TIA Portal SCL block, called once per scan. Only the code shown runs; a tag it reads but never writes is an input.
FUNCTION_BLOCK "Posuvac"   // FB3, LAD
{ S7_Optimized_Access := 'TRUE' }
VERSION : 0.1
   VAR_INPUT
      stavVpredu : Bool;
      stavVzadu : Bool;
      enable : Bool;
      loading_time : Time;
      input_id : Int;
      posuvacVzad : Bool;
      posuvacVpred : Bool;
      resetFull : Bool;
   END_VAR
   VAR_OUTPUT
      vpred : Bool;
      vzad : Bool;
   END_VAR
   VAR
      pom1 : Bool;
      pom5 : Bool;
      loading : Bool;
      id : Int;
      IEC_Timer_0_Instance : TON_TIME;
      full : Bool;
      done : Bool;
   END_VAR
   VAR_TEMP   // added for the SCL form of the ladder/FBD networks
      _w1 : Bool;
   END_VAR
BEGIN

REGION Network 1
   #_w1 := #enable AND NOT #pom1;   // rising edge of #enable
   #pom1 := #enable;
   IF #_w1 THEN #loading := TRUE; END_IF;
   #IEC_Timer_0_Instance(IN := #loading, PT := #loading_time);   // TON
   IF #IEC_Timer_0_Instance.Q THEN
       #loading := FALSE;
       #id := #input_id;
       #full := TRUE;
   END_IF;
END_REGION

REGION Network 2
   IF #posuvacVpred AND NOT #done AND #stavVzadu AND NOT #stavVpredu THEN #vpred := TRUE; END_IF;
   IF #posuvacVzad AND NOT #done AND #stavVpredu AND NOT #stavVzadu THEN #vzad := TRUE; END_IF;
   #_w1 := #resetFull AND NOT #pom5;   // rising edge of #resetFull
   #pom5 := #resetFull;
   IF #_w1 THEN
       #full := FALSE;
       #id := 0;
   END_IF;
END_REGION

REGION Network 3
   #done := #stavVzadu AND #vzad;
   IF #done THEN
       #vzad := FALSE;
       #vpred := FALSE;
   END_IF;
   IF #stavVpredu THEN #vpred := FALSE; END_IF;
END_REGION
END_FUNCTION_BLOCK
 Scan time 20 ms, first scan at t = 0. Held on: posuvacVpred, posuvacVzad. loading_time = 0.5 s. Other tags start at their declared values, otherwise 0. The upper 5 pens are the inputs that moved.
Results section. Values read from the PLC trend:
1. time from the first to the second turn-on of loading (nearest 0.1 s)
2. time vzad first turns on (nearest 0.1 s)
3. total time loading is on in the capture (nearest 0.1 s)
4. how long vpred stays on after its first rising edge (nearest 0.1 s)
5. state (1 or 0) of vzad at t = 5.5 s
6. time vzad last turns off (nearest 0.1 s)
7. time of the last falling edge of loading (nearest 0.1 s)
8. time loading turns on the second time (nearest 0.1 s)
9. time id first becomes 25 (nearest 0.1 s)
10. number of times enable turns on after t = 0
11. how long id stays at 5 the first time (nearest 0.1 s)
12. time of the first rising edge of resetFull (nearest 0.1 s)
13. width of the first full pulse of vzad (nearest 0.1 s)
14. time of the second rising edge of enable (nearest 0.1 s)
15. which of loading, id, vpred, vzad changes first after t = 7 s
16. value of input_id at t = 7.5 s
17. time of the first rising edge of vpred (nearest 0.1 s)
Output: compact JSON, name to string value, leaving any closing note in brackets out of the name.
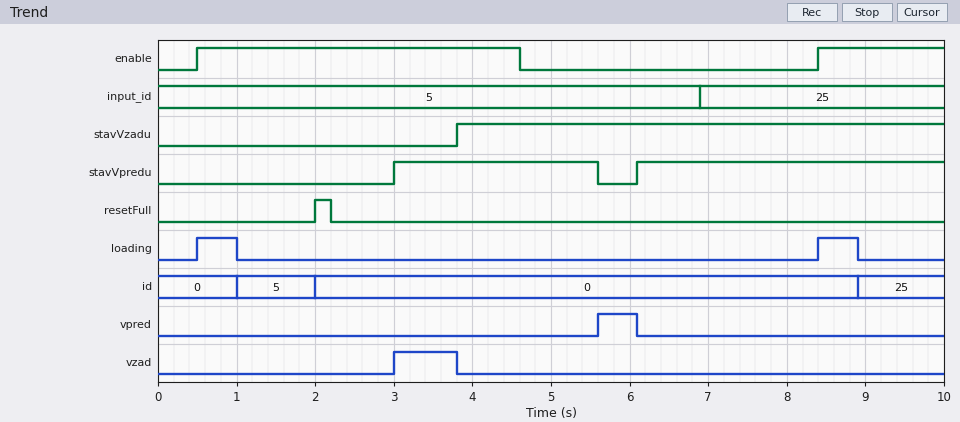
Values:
{"time from the first to the second turn-on of loading": "7.9 s", "time vzad first turns on": "3.0 s", "total time loading is on in the capture": "1.0 s", "how long vpred stays on after its first rising edge": "0.5 s", "state (1 or 0) of vzad at t = 5.5 s": "0", "time vzad last turns off": "3.8 s", "time of the last falling edge of loading": "8.9 s", "time loading turns on the second time": "8.4 s", "time id first becomes 25": "8.9 s", "number of times enable turns on after t = 0": "2", "how long id stays at 5 the first time": "1.0 s", "time of the first rising edge of resetFull": "2.0 s", "width of the first full pulse of vzad": "0.8 s", "time of the second rising edge of enable": "8.4 s", "which of loading, id, vpred, vzad changes first after t = 7 s": "loading", "value of input_id at t = 7.5 s": "25", "time of the first rising edge of vpred": "5.6 s"}
